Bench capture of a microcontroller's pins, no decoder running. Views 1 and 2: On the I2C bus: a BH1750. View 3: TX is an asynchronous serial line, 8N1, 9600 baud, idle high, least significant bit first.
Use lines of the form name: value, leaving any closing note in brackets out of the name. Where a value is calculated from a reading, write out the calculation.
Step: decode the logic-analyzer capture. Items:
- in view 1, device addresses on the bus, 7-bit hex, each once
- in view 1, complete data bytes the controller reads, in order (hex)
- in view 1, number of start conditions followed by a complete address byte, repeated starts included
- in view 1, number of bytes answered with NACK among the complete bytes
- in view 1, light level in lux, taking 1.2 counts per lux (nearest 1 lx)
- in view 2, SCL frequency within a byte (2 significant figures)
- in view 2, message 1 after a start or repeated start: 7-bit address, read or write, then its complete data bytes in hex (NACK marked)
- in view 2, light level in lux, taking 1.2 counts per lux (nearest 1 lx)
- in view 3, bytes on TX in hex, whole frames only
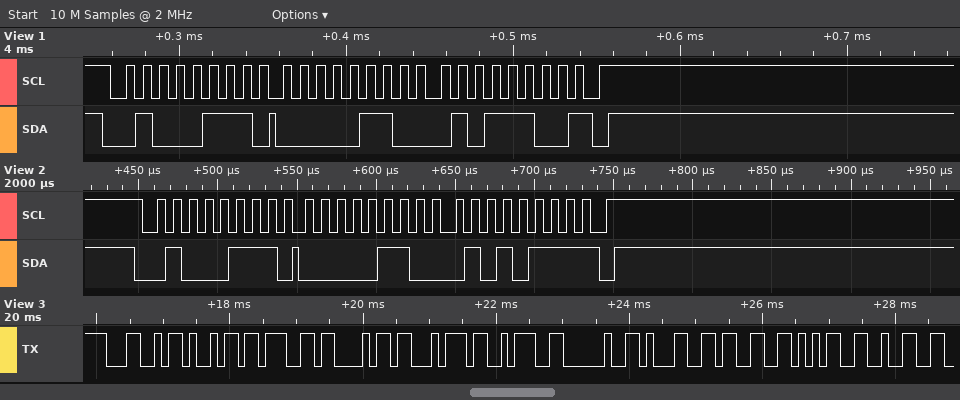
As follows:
in view 1, device addresses on the bus, 7-bit hex, each once: 0x23
in view 1, complete data bytes the controller reads, in order: 06 5C
in view 1, number of start conditions followed by a complete address byte, repeated starts included: 1
in view 1, number of bytes answered with NACK among the complete bytes: 1
in view 1, light level in lux, taking 1.2 counts per lux: 1628 / 1.2 = 1357 lx
in view 2, SCL frequency within a byte: 100 kHz
in view 2, message 1 after a start or repeated start: 7-bit address, read or write, then its complete data bytes in hex: 0x23 read: 06 57 NACK
in view 2, light level in lux, taking 1.2 counts per lux: 1623 / 1.2 = 1352 lx
in view 3, bytes on TX in hex, whole frames only: 4C 69 67 68 74 3A 20 31 33 35 32
